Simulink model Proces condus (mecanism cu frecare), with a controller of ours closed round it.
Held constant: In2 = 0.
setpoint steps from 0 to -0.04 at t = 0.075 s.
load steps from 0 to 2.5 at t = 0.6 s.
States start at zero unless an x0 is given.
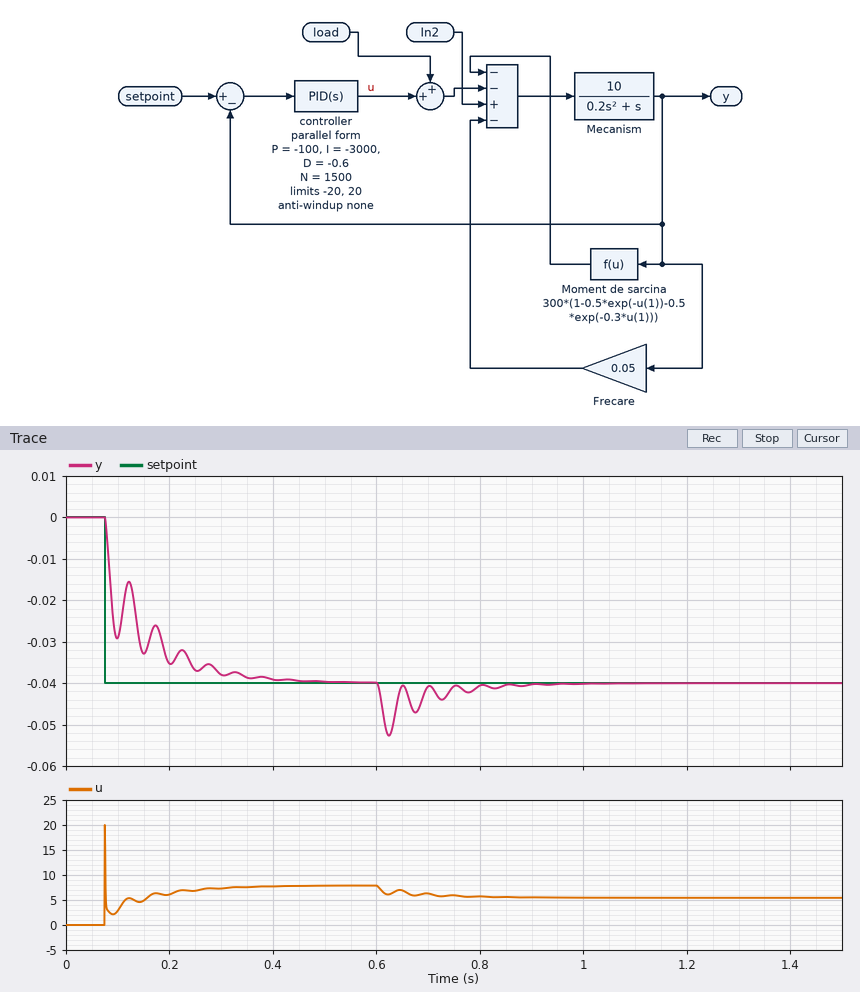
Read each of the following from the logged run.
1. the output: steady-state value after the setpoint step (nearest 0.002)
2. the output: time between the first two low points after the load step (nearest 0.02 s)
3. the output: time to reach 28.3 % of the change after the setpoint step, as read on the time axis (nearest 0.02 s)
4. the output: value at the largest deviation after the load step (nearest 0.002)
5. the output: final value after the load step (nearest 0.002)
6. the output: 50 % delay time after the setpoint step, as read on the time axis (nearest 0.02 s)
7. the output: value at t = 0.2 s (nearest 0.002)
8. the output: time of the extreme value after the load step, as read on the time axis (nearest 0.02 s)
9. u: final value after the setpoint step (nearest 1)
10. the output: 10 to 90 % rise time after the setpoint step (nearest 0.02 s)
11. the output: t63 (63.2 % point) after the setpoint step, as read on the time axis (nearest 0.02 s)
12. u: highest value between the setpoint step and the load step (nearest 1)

-0.040
0.06 s
0.08 s
-0.052
-0.040
0.08 s
-0.036
0.62 s
8
0.16 s
0.10 s
20
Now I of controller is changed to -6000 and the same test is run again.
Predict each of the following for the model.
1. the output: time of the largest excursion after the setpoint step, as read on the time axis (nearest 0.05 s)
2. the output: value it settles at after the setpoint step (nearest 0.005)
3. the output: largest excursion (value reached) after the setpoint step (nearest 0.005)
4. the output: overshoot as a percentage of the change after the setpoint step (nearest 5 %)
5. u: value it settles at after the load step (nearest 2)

0.20 s
-0.040
-0.045
10 %
6
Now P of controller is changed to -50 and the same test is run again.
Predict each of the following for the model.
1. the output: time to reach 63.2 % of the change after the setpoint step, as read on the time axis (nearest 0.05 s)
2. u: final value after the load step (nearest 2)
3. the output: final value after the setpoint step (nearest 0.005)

0.15 s
6
-0.040
